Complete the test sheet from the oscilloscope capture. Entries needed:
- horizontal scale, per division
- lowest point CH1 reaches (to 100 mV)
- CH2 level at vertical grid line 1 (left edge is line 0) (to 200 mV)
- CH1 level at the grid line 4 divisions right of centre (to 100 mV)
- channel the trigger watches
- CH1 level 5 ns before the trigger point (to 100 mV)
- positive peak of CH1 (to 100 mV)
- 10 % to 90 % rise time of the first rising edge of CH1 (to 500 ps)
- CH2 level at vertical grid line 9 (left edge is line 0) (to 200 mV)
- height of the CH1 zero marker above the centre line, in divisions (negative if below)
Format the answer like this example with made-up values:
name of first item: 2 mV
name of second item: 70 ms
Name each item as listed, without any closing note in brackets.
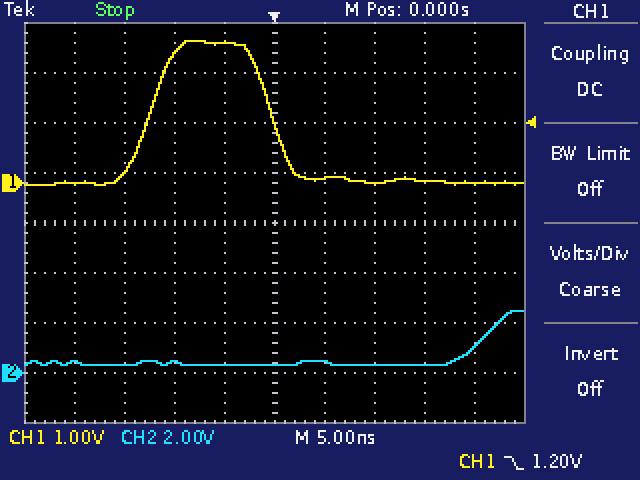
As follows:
horizontal scale, per division: 5 ns
lowest point CH1 reaches: 0.0 V
CH2 level at vertical grid line 1 (left edge is line 0): 400 mV
CH1 level at the grid line 4 divisions right of centre: 0.0 V
channel the trigger watches: CH1
CH1 level 5 ns before the trigger point: 2.8 V
positive peak of CH1: 2.8 V
10 % to 90 % rise time of the first rising edge of CH1: 4.5 ns
CH2 level at vertical grid line 9 (left edge is line 0): 1.0 V
height of the CH1 zero marker above the centre line, in divisions: +0.8 div
